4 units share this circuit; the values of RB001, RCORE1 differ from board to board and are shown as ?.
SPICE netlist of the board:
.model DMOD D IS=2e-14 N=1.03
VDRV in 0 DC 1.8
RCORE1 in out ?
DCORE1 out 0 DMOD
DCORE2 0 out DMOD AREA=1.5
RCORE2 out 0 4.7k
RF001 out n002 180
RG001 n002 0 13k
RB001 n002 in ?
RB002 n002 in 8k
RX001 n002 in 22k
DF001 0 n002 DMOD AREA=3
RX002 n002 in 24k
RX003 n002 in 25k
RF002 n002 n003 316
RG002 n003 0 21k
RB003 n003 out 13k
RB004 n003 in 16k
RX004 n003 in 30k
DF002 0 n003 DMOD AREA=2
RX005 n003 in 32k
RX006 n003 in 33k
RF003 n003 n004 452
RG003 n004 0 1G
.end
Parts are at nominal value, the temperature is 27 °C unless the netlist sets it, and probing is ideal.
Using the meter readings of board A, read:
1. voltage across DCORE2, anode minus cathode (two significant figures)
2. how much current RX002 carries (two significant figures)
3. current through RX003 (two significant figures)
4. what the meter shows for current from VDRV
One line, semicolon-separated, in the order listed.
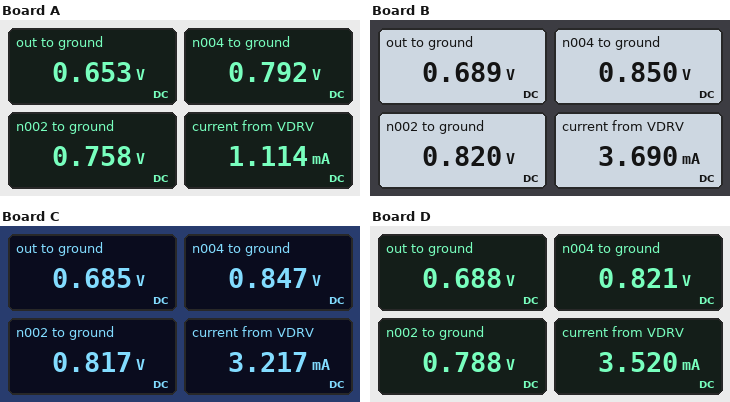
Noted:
-650 mV; 43 µA; 42 µA; 1.114 mA
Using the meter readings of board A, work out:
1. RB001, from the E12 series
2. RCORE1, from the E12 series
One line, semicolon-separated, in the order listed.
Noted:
3.9 kΩ; 2.7 kΩ
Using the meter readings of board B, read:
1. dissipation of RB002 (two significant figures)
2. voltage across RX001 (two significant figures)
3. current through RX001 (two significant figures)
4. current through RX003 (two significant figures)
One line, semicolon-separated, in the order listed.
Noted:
120 µW; 980 mV; 45 µA; 39 µA
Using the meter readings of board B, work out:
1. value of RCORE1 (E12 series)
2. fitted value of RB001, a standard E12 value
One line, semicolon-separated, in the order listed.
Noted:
390 Ω; 2.2 kΩ
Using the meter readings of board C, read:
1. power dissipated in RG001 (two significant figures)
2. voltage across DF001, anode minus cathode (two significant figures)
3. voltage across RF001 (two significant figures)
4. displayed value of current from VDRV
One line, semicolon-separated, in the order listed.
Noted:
51 µW; -820 mV; 130 mV; 3.217 mA
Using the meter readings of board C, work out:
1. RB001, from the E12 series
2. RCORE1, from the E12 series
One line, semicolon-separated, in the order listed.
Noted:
2.2 kΩ; 470 Ω
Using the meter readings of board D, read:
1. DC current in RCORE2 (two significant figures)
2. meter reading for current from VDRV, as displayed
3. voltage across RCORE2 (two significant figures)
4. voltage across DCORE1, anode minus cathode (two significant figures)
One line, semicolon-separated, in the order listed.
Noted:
150 µA; 3.520 mA; 690 mV; 690 mV
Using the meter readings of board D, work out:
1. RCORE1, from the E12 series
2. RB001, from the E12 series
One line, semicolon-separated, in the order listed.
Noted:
390 Ω; 3.9 kΩ
